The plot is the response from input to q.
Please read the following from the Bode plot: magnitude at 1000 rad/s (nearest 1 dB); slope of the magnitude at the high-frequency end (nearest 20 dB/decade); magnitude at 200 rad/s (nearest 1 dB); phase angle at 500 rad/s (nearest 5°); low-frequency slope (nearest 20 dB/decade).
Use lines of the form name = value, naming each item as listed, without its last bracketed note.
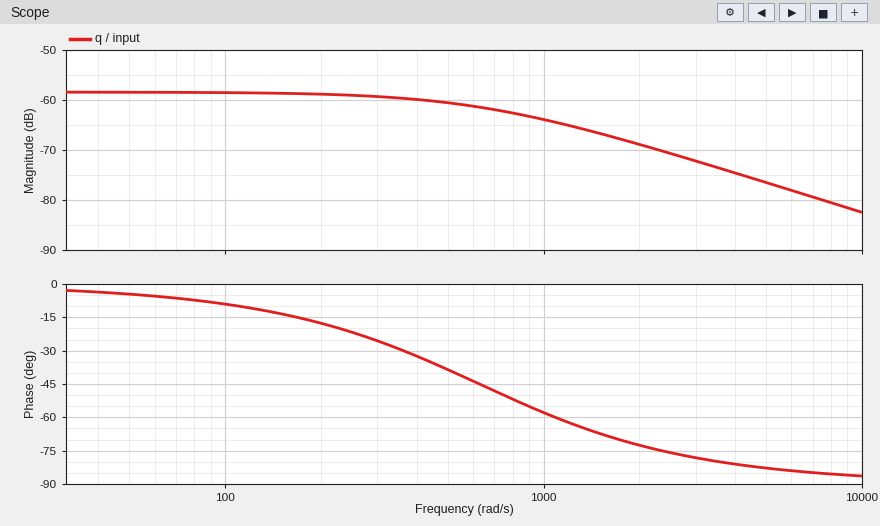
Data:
magnitude at 1000 rad/s = -64 dB
slope of the magnitude at the high-frequency end = -20 dB/decade
magnitude at 200 rad/s = -59 dB
phase angle at 500 rad/s = -40°
low-frequency slope = 0 dB/decade
